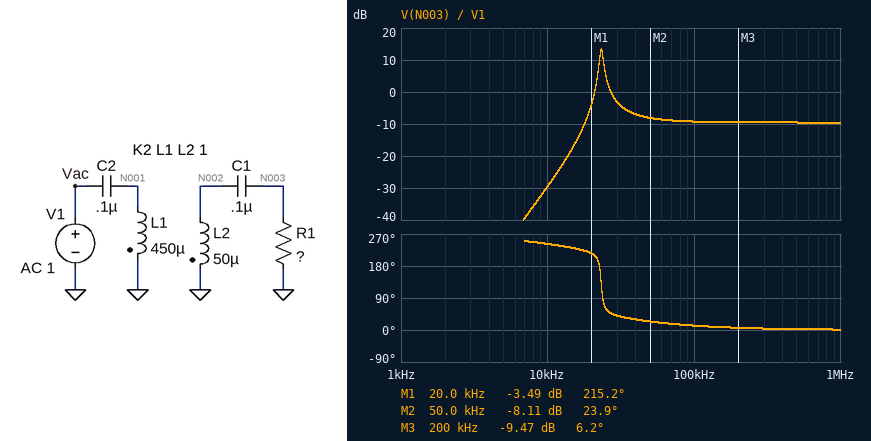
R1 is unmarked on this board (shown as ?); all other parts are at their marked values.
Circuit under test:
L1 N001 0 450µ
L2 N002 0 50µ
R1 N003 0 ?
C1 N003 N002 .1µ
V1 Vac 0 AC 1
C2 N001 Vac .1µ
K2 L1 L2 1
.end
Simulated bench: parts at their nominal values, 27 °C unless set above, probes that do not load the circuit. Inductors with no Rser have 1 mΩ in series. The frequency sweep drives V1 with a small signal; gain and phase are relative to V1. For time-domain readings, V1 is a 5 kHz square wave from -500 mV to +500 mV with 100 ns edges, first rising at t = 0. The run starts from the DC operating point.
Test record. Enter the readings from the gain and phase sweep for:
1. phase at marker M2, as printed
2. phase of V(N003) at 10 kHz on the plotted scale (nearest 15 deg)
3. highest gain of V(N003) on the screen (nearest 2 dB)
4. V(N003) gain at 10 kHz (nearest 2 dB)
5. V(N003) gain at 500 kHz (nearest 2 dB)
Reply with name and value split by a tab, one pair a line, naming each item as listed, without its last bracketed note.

phase at marker M2, as printed	23.9 deg
phase of V(N003) at 10 kHz on the plotted scale	240 deg
highest gain of V(N003) on the screen	14 dB
V(N003) gain at 10 kHz	-30 dB
V(N003) gain at 500 kHz	-10 dB
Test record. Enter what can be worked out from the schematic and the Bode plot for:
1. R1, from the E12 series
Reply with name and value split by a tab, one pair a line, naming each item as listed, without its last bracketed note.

R1, from the E12 series	82 Ω
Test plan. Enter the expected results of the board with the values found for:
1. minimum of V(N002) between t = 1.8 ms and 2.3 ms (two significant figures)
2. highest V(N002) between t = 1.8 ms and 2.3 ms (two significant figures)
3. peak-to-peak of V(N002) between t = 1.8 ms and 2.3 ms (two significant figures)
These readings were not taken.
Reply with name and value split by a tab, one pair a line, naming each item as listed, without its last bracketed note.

minimum of V(N002) between t = 1.8 ms and 2.3 ms	-340 mV
highest V(N002) between t = 1.8 ms and 2.3 ms	340 mV
peak-to-peak of V(N002) between t = 1.8 ms and 2.3 ms	680 mV
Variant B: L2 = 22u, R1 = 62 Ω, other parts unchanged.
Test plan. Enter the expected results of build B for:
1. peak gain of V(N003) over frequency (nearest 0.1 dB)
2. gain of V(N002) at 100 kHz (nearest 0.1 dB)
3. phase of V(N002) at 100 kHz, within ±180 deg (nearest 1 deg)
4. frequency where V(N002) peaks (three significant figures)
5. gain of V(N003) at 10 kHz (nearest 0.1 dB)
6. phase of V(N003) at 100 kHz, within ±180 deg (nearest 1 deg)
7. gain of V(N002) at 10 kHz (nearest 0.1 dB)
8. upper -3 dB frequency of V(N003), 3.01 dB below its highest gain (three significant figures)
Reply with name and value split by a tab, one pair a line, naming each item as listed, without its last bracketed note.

peak gain of V(N003) over frequency	15.7 dB
gain of V(N002) at 100 kHz	-12.6 dB
phase of V(N002) at 100 kHz, within ±180 deg	1 deg
frequency where V(N002) peaks	23.4 kHz
gain of V(N003) at 10 kHz	-35.1 dB
phase of V(N003) at 100 kHz, within ±180 deg	15 deg
gain of V(N002) at 10 kHz	-26.3 dB
upper -3 dB frequency of V(N003), 3.01 dB below its highest gain	23.7 kHz
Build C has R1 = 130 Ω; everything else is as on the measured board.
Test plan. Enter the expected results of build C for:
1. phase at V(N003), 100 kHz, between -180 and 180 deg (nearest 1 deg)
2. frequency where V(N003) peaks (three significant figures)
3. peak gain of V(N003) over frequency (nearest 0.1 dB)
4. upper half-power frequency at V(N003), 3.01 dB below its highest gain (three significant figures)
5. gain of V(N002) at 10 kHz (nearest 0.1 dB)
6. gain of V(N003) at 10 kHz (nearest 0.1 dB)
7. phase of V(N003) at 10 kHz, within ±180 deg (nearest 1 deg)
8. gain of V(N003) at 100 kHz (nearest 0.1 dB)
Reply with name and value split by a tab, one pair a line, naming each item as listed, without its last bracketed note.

phase at V(N003), 100 kHz, between -180 and 180 deg	8 deg
frequency where V(N003) peaks	23.5 kHz
peak gain of V(N003) over frequency	16.2 dB
upper half-power frequency at V(N003), 3.01 dB below its highest gain	24.0 kHz
gain of V(N002) at 10 kHz	-22.7 dB
gain of V(N003) at 10 kHz	-26.7 dB
phase of V(N003) at 10 kHz, within ±180 deg	-130 deg
gain of V(N003) at 100 kHz	-9.1 dB
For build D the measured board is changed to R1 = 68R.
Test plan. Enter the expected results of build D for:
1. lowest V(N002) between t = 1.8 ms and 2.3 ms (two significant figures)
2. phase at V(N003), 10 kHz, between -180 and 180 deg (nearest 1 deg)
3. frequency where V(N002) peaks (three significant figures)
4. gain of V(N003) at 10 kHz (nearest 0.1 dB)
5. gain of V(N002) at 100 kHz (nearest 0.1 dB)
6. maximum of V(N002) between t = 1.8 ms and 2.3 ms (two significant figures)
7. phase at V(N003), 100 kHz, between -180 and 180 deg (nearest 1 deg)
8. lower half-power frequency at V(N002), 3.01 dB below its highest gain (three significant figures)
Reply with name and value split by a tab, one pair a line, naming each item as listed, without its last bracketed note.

lowest V(N002) between t = 1.8 ms and 2.3 ms	-320 mV
phase at V(N003), 10 kHz, between -180 and 180 deg	-114 deg
frequency where V(N002) peaks	23.1 kHz
gain of V(N003) at 10 kHz	-30.8 dB
gain of V(N002) at 100 kHz	-9.1 dB
maximum of V(N002) between t = 1.8 ms and 2.3 ms	320 mV
phase at V(N003), 100 kHz, between -180 and 180 deg	15 deg
lower half-power frequency at V(N002), 3.01 dB below its highest gain	22.5 kHz
